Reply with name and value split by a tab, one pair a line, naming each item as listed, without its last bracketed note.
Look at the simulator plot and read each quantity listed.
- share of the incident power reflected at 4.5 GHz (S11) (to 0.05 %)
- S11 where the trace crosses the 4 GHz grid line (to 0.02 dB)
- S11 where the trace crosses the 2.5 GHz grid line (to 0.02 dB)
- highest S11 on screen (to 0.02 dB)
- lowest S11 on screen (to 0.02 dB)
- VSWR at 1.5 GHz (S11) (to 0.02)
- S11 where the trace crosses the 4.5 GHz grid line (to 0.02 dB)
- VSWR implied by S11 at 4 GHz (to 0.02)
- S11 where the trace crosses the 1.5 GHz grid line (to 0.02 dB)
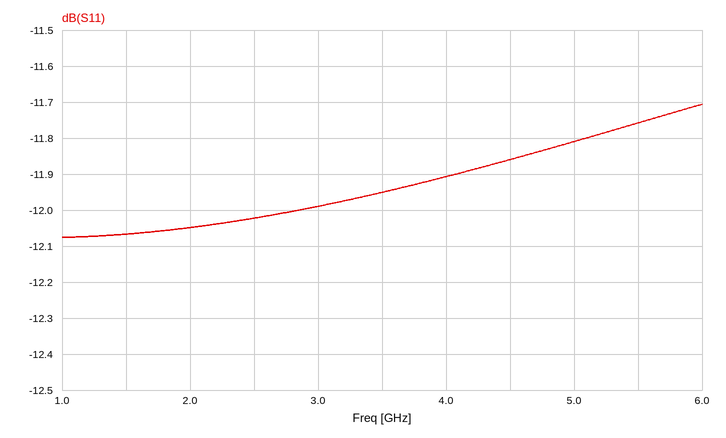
share of the incident power reflected at 4.5 GHz (S11)	6.50 %
S11 where the trace crosses the 4 GHz grid line	-11.90 dB
S11 where the trace crosses the 2.5 GHz grid line	-12.02 dB
highest S11 on screen	-11.70 dB
lowest S11 on screen	-12.08 dB
VSWR at 1.5 GHz (S11)	1.66
S11 where the trace crosses the 4.5 GHz grid line	-11.86 dB
VSWR implied by S11 at 4 GHz	1.68
S11 where the trace crosses the 1.5 GHz grid line	-12.06 dB
